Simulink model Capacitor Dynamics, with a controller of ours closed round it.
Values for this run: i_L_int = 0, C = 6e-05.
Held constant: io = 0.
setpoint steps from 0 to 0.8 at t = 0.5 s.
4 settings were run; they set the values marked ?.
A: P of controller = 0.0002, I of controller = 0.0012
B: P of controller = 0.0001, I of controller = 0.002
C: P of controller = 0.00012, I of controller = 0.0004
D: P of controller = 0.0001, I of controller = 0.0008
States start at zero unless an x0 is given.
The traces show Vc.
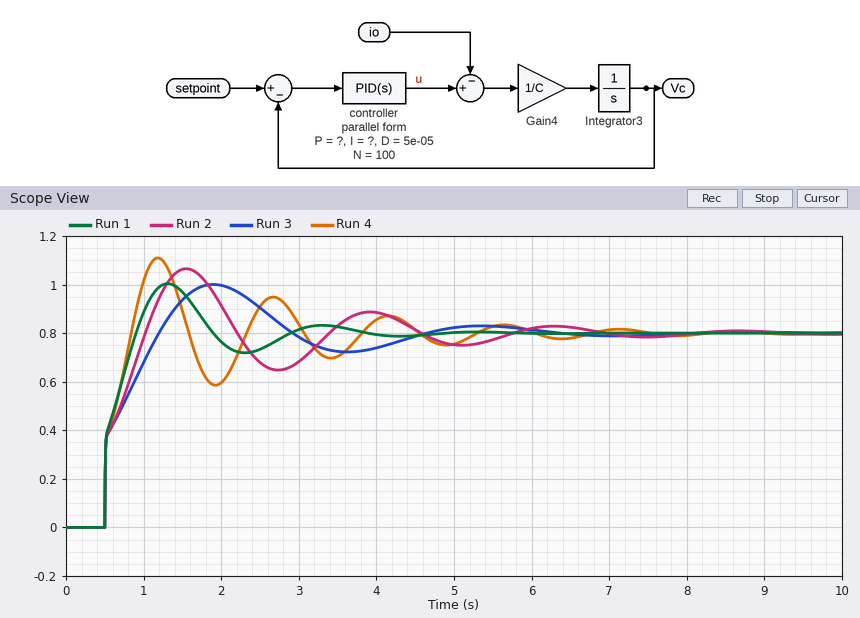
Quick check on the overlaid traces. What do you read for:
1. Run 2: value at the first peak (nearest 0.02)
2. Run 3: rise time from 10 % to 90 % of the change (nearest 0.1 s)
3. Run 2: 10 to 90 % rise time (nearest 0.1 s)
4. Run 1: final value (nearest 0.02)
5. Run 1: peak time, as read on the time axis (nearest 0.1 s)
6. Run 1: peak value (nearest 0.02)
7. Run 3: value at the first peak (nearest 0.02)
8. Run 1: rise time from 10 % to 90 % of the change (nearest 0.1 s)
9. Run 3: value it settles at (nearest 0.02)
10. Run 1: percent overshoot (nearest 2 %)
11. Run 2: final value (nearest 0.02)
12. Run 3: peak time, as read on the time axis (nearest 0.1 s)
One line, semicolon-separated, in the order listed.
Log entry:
1.06; 0.6 s; 0.4 s; 0.80; 1.3 s; 1.00; 1.00; 0.3 s; 0.80; 26 %; 0.80; 1.9 s
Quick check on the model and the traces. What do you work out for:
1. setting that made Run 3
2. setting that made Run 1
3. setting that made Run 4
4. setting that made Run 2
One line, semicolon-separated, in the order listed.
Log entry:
C; A; B; D
